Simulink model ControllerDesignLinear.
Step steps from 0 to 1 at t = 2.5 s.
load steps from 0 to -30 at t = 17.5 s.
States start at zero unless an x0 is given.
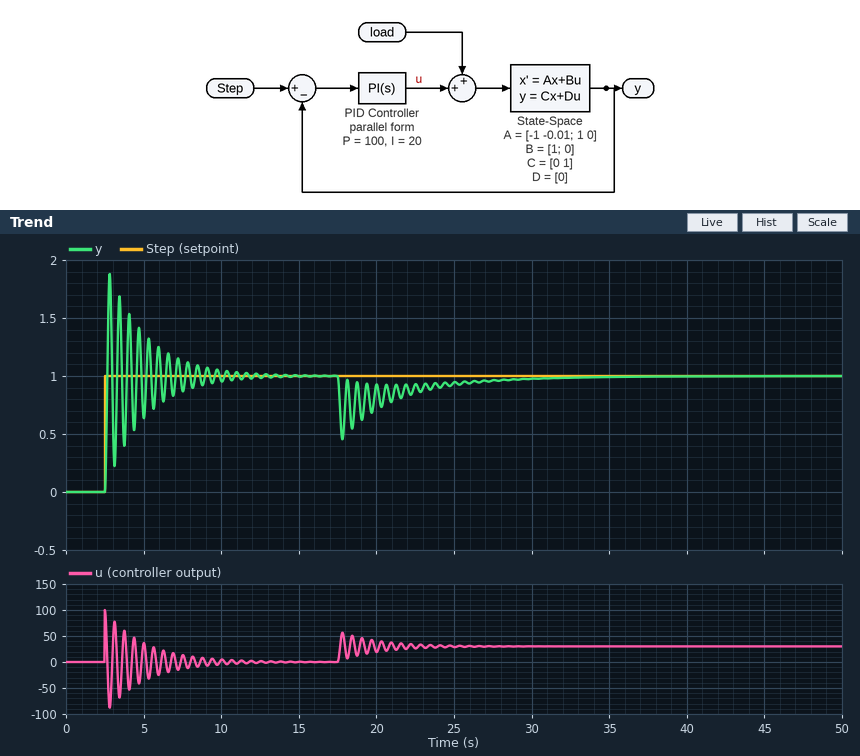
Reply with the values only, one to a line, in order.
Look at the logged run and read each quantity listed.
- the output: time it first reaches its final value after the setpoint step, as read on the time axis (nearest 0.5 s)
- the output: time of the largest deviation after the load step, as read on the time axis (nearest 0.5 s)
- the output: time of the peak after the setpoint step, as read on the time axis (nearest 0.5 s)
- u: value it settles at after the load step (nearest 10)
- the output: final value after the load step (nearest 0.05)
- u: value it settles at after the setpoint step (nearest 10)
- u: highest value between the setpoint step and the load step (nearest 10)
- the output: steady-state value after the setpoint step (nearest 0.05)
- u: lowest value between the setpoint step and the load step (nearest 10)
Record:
2.5 s
18.0 s
3.0 s
30
1.00
0
100
1.00
-90
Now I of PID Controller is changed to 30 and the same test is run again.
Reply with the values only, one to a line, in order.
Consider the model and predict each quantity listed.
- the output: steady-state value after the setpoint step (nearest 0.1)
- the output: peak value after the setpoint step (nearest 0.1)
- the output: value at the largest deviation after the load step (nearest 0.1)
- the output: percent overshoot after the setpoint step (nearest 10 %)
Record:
1.0
1.9
0.5
90 %
